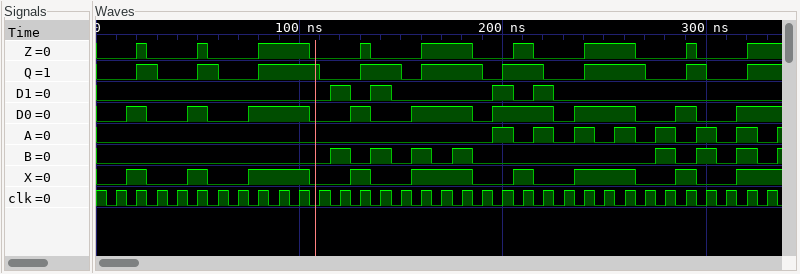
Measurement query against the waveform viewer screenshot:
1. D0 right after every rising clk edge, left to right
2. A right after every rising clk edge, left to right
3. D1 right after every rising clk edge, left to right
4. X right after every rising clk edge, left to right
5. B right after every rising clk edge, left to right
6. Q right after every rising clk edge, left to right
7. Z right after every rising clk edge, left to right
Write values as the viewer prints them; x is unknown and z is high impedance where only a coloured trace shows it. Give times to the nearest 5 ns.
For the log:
0 1 0 0 1 0 0 1 1 1 0 0 1 0 0 1 1 1 0 1 1 1 0 1 1 1 0 0 1 0 0 1 1
0 0 0 0 0 0 0 0 0 0 0 0 0 0 0 0 0 0 0 1 0 1 0 1 0 1 0 1 0 1 0 1 0
0 0 0 0 0 0 0 0 0 0 0 1 0 1 0 0 0 0 0 1 0 1 0 0 0 0 0 0 0 0 0 0 0
0 1 0 0 1 0 0 1 1 1 0 0 1 0 0 1 1 1 0 0 1 0 0 1 1 1 0 0 1 0 0 1 1
0 0 0 0 0 0 0 0 0 0 0 1 0 1 0 1 0 1 0 0 0 0 0 0 0 0 0 1 0 1 0 1 0
0 1 0 0 1 0 0 1 1 1 0 0 1 1 0 1 1 1 0 1 1 0 0 1 1 1 0 0 1 0 0 1 1
0 1 0 0 1 0 0 1 1 1 0 0 1 0 0 1 1 1 0 0 1 0 0 1 1 1 0 0 1 0 0 1 1
